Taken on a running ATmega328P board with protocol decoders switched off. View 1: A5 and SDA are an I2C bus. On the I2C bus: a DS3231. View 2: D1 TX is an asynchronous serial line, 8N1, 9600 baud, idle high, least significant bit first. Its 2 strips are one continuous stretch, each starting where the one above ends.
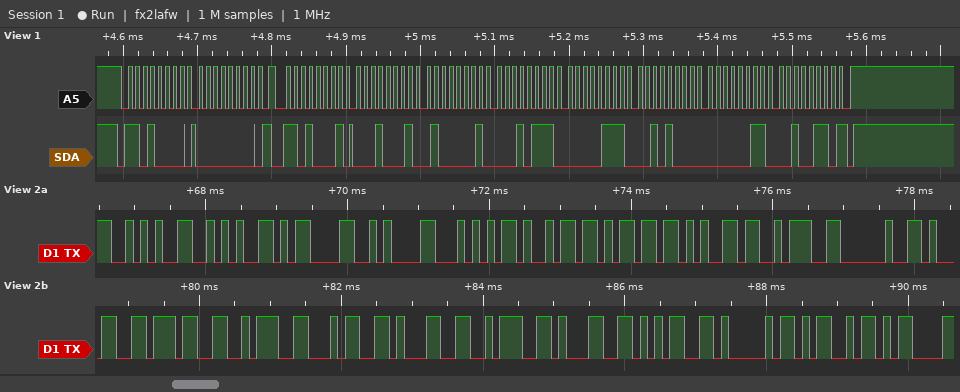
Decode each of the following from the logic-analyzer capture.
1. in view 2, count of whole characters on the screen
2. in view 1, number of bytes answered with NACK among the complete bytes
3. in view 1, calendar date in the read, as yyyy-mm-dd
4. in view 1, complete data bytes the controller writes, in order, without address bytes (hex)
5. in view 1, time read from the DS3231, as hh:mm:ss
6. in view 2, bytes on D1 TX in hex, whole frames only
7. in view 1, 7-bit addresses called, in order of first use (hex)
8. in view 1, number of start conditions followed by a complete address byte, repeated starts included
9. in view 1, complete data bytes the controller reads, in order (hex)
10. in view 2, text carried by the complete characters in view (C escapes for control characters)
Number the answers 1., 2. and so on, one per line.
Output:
1. 21
2. 1
3. 2026-03-28
4. 00
5. 17:41:11
6. 2A 2A 0D 0A 54 69 6D 65 3A 20 31 37 3A 34 31 3A 31 35 41 4D 0D
7. 0x68
8. 2
9. 11 41 17 07 28 03 26
10. "**\r\nTime: 17:41:15AM\r"
